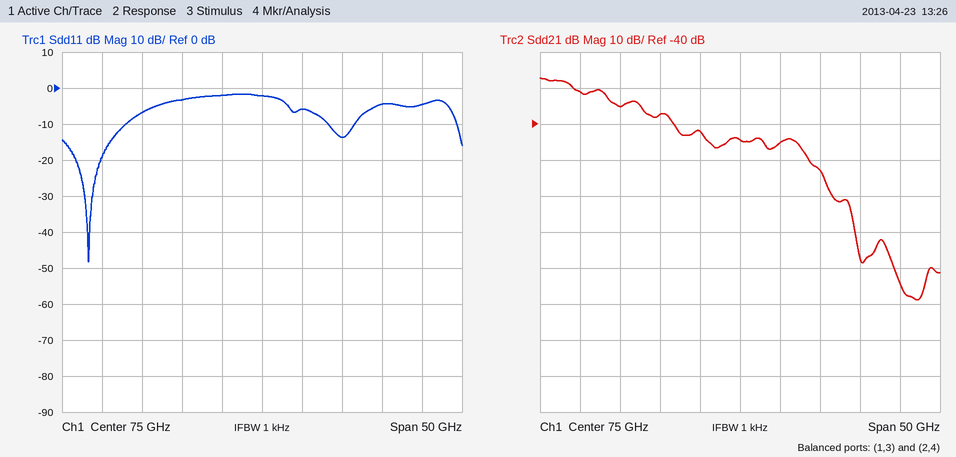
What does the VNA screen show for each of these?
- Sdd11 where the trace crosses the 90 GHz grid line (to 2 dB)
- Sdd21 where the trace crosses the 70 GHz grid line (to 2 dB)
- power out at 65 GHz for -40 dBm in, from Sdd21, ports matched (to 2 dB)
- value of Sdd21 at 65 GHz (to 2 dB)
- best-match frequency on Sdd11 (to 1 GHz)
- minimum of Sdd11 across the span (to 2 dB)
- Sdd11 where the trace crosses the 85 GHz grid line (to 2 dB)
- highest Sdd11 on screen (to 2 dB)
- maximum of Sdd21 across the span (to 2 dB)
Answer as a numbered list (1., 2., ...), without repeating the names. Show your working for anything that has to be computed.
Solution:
1. -4 dB
2. -42 dB
3. -40 dBm + (-38 dB) = -78 dBm
4. -38 dB
5. 53 GHz
6. -48 dB
7. -14 dB
8. -2 dB
9. -28 dB
